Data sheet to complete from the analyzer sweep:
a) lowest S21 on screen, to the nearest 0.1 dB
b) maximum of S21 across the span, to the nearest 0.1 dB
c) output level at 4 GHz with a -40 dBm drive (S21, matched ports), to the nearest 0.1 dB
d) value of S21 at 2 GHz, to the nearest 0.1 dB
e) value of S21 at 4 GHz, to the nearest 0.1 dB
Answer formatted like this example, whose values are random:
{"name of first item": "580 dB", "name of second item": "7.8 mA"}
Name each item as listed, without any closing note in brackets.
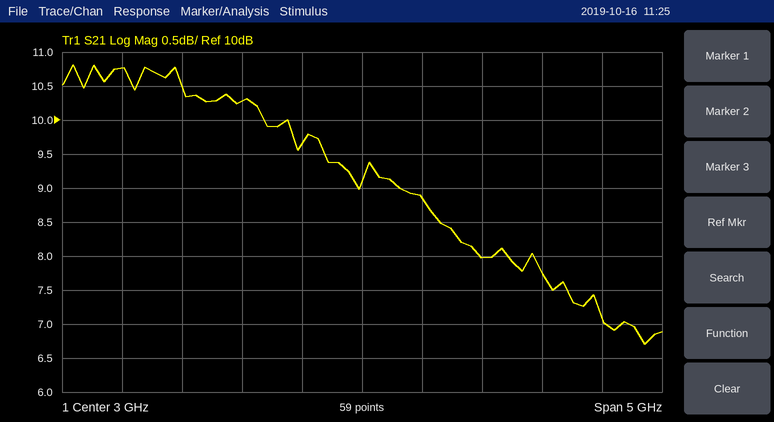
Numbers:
{"lowest S21 on screen, to the nearest 0.1 dB": "6.7 dB", "maximum of S21 across the span, to the nearest 0.1 dB": "10.8 dB", "output level at 4 GHz with a -40 dBm drive (S21, matched ports), to the nearest 0.1 dB": "-32.0 dBm", "value of S21 at 2 GHz, to the nearest 0.1 dB": "10.3 dB", "value of S21 at 4 GHz, to the nearest 0.1 dB": "8.0 dB"}
